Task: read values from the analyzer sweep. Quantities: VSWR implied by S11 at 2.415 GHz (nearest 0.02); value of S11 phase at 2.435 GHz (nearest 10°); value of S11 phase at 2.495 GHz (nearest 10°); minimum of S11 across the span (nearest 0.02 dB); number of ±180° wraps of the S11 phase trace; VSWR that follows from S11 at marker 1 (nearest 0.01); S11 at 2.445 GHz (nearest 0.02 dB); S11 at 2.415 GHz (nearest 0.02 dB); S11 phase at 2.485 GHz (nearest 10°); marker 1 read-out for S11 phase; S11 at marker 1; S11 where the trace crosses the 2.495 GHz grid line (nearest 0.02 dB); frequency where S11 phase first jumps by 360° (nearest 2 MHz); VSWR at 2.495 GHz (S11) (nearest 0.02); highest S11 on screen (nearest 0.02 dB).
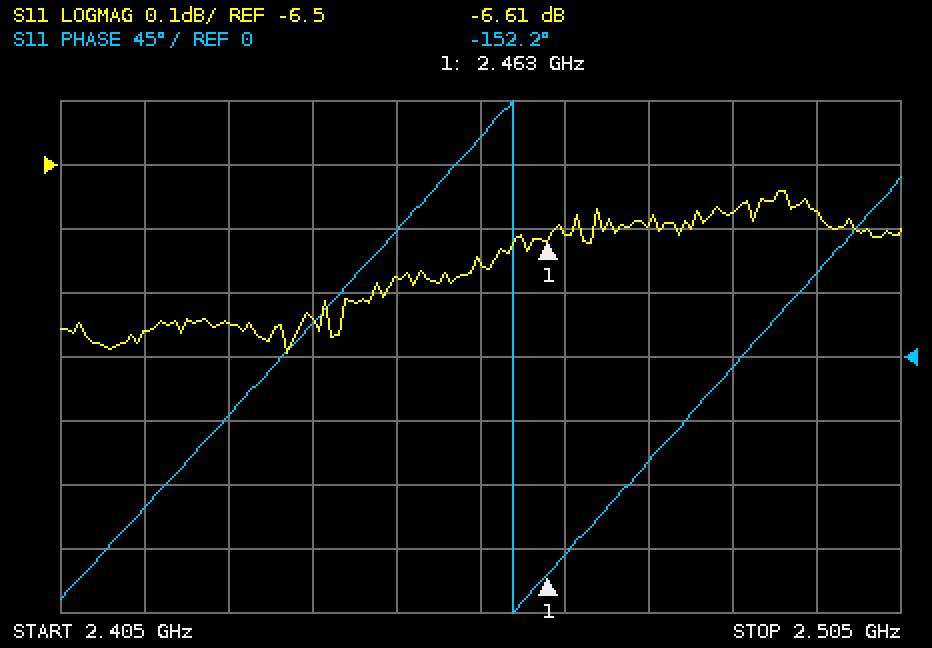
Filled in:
2.70
20°
60°
-6.80 dB
1
2.75
-6.68 dB
-6.76 dB
-10°
-152.2°
-6.61 dB
-6.58 dB
2.458 GHz
2.76
-6.54 dB
